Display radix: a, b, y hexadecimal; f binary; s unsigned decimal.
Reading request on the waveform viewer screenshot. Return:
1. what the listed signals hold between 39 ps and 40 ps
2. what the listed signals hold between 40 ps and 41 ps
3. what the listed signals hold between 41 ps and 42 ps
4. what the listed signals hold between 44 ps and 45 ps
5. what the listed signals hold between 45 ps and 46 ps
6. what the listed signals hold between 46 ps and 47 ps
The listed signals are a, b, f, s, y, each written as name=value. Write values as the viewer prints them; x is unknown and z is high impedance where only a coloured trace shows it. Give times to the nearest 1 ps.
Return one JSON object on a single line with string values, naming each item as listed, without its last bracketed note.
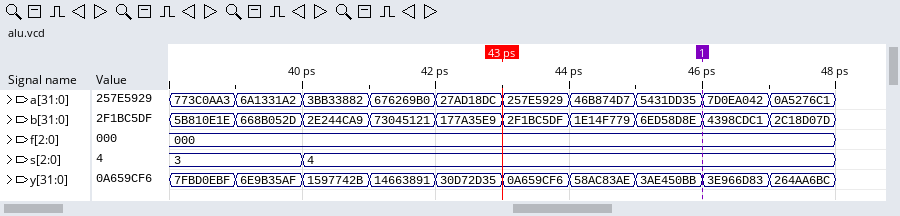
{"what the listed signals hold between 39 ps and 40 ps": "a=6A1331A2, b=668B052D, f=000, s=3, y=6E9B35AF", "what the listed signals hold between 40 ps and 41 ps": "a=3BB33882, b=2E244CA9, f=000, s=4, y=1597742B", "what the listed signals hold between 41 ps and 42 ps": "a=676269B0, b=73045121, f=000, s=4, y=14663891", "what the listed signals hold between 44 ps and 45 ps": "a=46B874D7, b=1E14F779, f=000, s=4, y=58AC83AE", "what the listed signals hold between 45 ps and 46 ps": "a=5431DD35, b=6ED58D8E, f=000, s=4, y=3AE450BB", "what the listed signals hold between 46 ps and 47 ps": "a=7D0EA042, b=4398CDC1, f=000, s=4, y=3E966D83"}
